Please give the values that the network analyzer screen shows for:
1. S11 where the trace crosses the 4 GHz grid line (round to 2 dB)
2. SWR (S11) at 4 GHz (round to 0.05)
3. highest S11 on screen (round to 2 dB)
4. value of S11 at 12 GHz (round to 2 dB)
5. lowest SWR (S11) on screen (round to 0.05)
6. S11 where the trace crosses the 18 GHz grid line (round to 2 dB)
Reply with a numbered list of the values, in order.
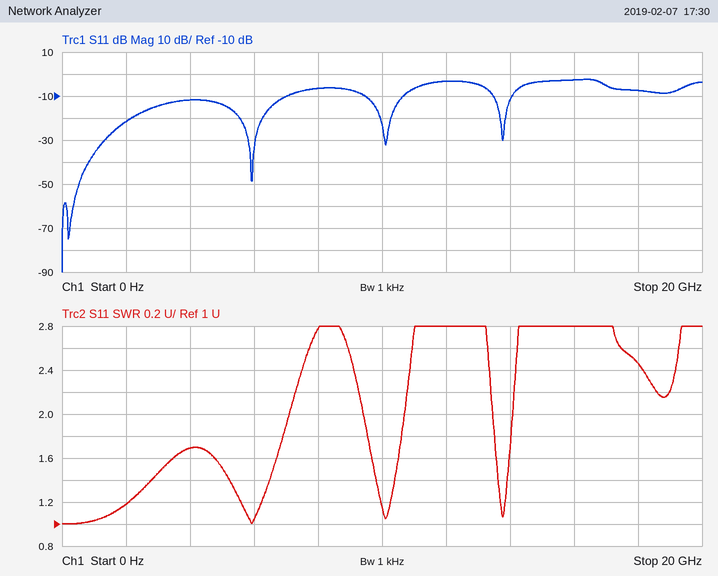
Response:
1. -12 dB
2. 1.70
3. -2 dB
4. -4 dB
5. 1.00
6. -8 dB
